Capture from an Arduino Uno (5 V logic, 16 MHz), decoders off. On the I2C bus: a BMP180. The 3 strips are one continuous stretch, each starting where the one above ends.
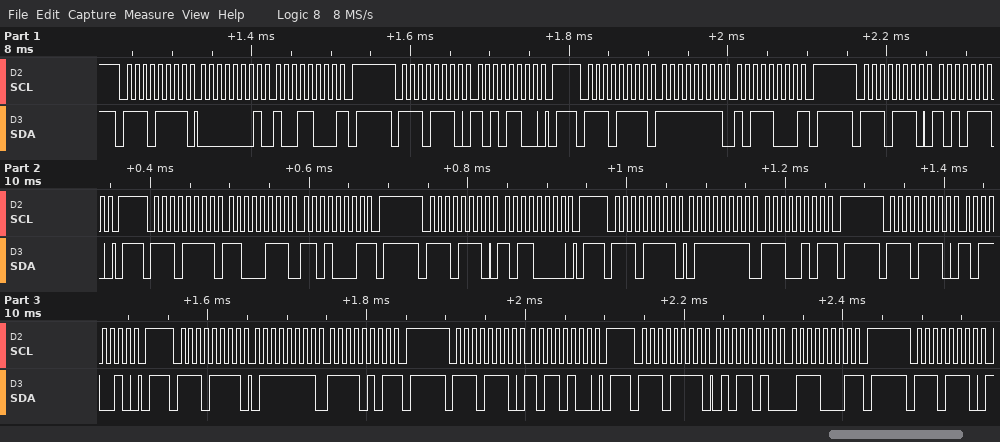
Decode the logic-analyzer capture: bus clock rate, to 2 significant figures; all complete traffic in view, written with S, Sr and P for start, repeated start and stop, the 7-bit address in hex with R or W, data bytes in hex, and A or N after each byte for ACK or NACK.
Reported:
100 kHz
S 77R A 01 A 98 N P S 77W A AC A P S 77R A FF A B8 N P S 77W A AE A P S 77R A C7 A D1 N P S 77W A B0 A P S 77R A 7F A E5 N P S 77W A B2 A P S 77R A 7F A F5 N P S 77W A B4 A P S 77R A 5A A 71 N P S 77W A
